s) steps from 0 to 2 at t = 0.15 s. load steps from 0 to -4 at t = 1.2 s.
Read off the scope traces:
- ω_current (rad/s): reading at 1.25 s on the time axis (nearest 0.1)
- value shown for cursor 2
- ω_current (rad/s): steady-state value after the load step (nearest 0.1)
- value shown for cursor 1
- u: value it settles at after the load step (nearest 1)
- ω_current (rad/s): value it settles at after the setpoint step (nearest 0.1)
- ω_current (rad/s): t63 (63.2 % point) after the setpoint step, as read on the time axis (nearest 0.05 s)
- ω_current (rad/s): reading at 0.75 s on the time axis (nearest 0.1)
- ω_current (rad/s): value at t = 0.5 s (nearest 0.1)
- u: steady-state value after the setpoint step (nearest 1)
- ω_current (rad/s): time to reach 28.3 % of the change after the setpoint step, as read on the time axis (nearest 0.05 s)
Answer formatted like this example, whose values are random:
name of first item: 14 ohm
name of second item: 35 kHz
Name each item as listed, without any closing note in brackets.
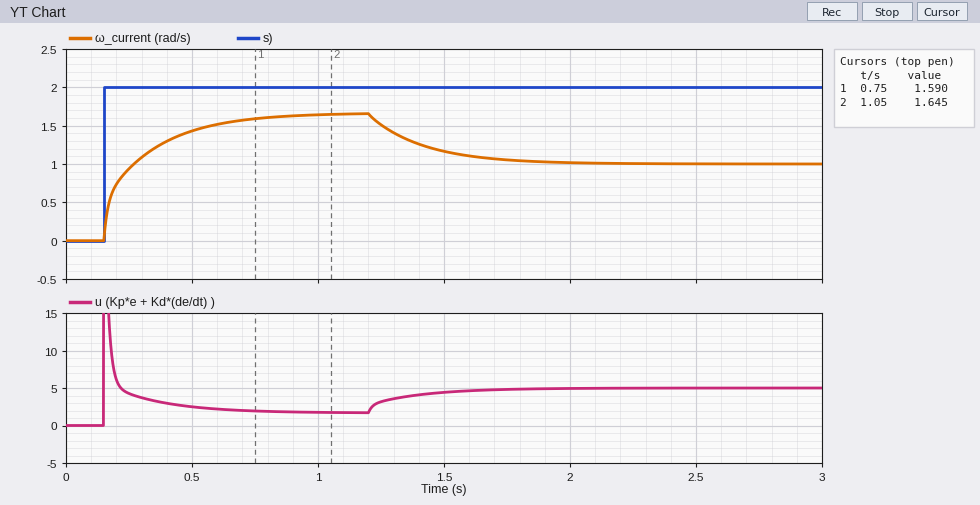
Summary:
ω_current (rad/s): reading at 1.25 s on the time axis: 1.5
value shown for cursor 2: 1.645
ω_current (rad/s): steady-state value after the load step: 1.0
value shown for cursor 1: 1.590
u: value it settles at after the load step: 5
ω_current (rad/s): value it settles at after the setpoint step: 1.7
ω_current (rad/s): t63 (63.2 % point) after the setpoint step, as read on the time axis: 0.30 s
ω_current (rad/s): reading at 0.75 s on the time axis: 1.6
ω_current (rad/s): value at t = 0.5 s: 1.4
u: steady-state value after the setpoint step: 2
ω_current (rad/s): time to reach 28.3 % of the change after the setpoint step, as read on the time axis: 0.15 s
